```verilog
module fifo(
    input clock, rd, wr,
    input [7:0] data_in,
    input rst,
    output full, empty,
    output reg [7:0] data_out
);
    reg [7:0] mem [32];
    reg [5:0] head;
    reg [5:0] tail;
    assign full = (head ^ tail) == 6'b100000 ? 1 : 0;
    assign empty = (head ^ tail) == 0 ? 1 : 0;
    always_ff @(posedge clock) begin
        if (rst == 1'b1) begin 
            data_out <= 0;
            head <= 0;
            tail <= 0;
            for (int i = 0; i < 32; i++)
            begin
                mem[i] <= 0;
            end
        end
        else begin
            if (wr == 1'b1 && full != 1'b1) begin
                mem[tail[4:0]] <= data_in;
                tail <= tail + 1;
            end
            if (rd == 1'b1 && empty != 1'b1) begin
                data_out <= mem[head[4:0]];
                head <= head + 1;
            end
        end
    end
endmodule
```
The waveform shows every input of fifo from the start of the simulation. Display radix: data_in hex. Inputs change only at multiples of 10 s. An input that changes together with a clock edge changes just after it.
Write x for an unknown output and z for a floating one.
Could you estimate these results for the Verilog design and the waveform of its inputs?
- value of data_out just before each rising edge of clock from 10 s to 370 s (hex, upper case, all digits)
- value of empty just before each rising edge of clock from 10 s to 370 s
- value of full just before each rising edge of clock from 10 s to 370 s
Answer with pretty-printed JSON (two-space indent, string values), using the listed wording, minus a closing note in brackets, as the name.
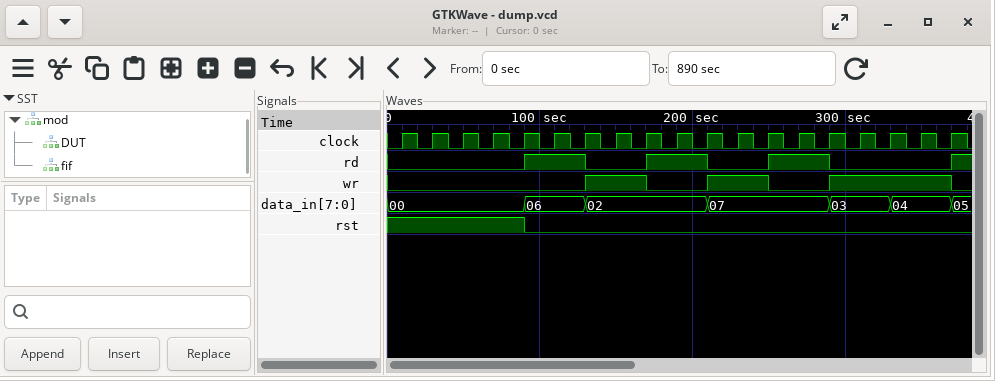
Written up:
{
  "value of data_out just before each rising edge of clock from 10 s to 370 s": "x, 00, 00, 00, 00, 00, 00, 00, 00, 00, 02, 02, 02, 02, 07, 07, 07, 07, 07",
  "value of empty just before each rising edge of clock from 10 s to 370 s": "x 1 1 1 1 1 1 1 0 0 0 1 0 0 0 1 0 0 0",
  "value of full just before each rising edge of clock from 10 s to 370 s": "x 0 0 0 0 0 0 0 0 0 0 0 0 0 0 0 0 0 0"
}
